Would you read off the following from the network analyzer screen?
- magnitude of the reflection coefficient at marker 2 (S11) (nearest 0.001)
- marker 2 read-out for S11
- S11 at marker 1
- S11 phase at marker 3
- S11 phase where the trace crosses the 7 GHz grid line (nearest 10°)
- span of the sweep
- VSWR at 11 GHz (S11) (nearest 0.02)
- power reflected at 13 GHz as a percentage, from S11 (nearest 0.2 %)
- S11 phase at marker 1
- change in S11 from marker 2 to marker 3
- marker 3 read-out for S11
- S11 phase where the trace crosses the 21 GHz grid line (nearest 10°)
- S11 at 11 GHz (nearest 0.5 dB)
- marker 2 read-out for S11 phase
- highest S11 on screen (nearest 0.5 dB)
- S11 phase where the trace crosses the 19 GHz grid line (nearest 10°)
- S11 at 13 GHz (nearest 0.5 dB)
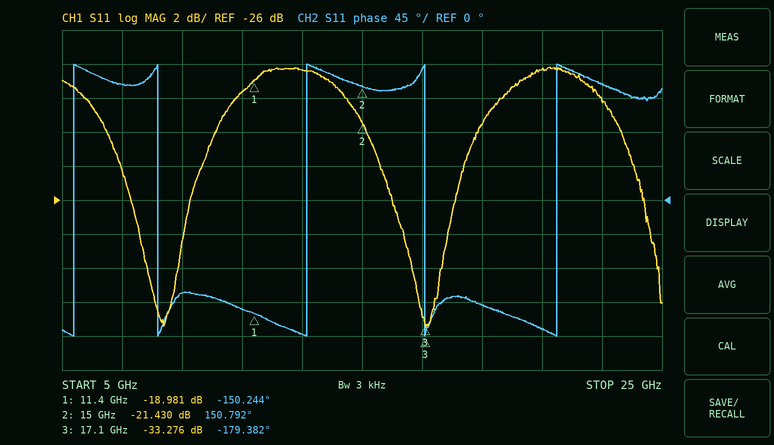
0.085
-21.430 dB
-18.981 dB
-179.382°
150°
20 GHz
1.24
1.4 %
-150.244°
-11.846 dB
-33.276 dB
-170°
-19.5 dB
150.792°
-18.0 dB
-140°
-18.5 dB
